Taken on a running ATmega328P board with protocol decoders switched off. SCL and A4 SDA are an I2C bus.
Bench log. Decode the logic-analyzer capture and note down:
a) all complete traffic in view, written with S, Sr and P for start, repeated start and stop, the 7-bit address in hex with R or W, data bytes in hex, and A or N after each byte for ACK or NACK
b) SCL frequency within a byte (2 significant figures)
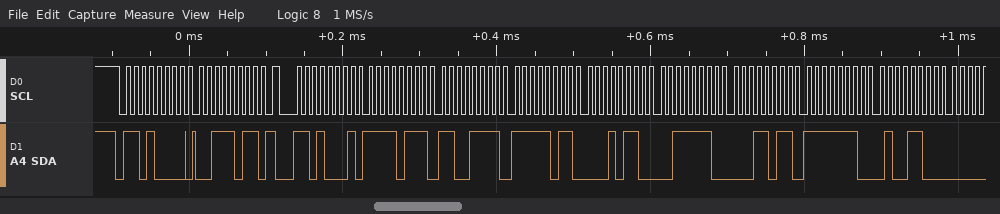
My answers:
S 68W A 3B A Sr 68R A F7 A CF A FB A 16 A 3E A 1B A FE A 4C A
100 kHz
